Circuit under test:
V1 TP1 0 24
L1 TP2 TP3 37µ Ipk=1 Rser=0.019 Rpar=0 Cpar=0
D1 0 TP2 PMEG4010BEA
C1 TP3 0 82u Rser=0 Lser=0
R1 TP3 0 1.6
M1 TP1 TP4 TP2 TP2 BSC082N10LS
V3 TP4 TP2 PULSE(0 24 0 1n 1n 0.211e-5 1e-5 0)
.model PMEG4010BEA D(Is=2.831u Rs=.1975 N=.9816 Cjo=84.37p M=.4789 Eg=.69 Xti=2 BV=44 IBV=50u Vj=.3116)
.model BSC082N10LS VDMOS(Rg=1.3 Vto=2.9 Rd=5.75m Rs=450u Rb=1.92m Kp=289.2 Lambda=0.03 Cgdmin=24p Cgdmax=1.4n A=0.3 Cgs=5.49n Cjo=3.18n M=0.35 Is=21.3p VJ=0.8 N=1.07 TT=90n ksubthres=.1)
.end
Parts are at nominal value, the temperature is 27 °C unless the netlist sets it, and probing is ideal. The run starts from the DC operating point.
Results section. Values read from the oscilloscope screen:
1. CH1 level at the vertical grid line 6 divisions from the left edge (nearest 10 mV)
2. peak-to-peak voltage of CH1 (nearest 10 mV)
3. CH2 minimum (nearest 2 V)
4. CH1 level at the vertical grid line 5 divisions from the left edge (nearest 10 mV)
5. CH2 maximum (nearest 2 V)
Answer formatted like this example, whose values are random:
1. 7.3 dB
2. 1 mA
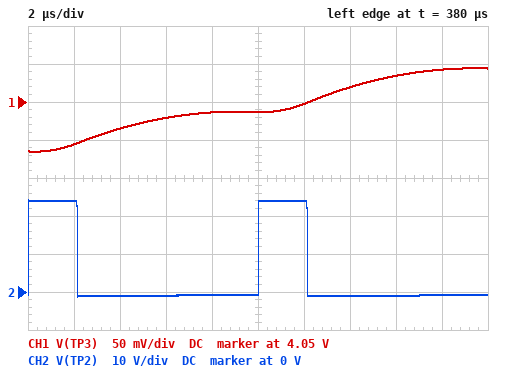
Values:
1. 4.05 V
2. 110 mV
3. -2 V
4. 4.04 V
5. 24 V
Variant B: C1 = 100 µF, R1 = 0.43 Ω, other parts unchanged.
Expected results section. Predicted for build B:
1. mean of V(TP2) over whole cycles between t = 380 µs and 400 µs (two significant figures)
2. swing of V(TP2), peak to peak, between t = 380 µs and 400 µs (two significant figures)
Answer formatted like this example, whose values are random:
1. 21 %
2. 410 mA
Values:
1. 3.6 V
2. 26 V
